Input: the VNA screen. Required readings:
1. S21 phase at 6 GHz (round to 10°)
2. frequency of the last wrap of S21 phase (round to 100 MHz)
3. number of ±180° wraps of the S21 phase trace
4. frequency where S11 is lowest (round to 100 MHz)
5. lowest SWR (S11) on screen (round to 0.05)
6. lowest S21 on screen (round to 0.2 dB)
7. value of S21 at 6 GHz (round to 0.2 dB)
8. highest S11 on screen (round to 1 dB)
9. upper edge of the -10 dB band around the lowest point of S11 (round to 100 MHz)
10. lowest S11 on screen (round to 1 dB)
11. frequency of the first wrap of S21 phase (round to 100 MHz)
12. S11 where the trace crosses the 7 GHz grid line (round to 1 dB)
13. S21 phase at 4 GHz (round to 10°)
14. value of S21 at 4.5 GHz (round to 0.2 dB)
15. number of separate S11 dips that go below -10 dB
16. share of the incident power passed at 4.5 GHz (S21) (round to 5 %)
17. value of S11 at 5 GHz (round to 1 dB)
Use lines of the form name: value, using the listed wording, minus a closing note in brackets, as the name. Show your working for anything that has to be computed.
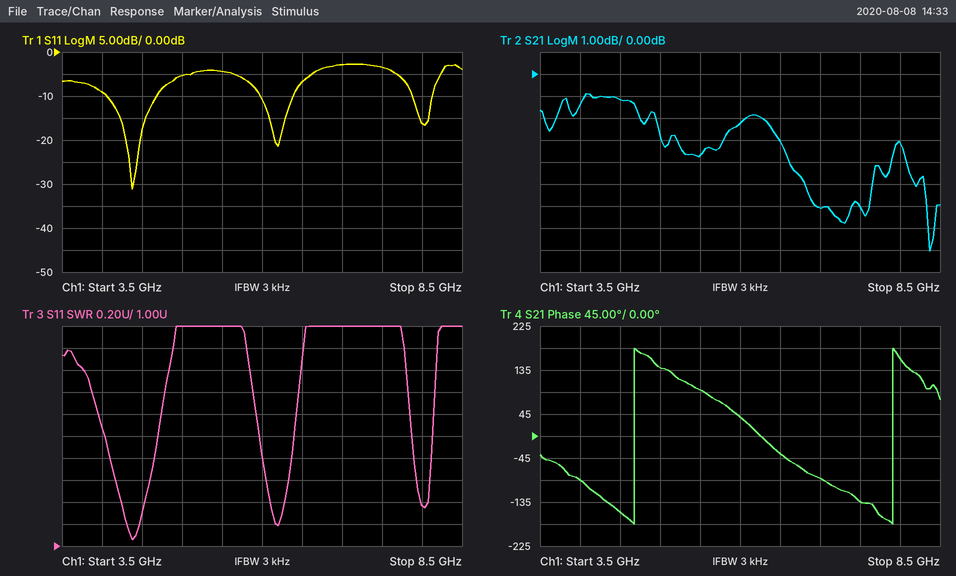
S21 phase at 6 GHz: 40°
frequency of the last wrap of S21 phase: 7.9 GHz
number of ±180° wraps of the S21 phase trace: 2
frequency where S11 is lowest: 4.4 GHz
lowest SWR (S11) on screen: 1.05
lowest S21 on screen: -8.0 dB
value of S21 at 6 GHz: -2.2 dB
highest S11 on screen: -3 dB
upper edge of the -10 dB band around the lowest point of S11: 4.7 GHz
lowest S11 on screen: -31 dB
frequency of the first wrap of S21 phase: 4.7 GHz
S11 where the trace crosses the 7 GHz grid line: -3 dB
S21 phase at 4 GHz: -90°
value of S21 at 4.5 GHz: -1.2 dB
number of separate S11 dips that go below -10 dB: 3
share of the incident power passed at 4.5 GHz (S21): 10^(-1.2/10) ≈ 75.9 %, so 75 % to the nearest 5 %
value of S11 at 5 GHz: -5 dB
